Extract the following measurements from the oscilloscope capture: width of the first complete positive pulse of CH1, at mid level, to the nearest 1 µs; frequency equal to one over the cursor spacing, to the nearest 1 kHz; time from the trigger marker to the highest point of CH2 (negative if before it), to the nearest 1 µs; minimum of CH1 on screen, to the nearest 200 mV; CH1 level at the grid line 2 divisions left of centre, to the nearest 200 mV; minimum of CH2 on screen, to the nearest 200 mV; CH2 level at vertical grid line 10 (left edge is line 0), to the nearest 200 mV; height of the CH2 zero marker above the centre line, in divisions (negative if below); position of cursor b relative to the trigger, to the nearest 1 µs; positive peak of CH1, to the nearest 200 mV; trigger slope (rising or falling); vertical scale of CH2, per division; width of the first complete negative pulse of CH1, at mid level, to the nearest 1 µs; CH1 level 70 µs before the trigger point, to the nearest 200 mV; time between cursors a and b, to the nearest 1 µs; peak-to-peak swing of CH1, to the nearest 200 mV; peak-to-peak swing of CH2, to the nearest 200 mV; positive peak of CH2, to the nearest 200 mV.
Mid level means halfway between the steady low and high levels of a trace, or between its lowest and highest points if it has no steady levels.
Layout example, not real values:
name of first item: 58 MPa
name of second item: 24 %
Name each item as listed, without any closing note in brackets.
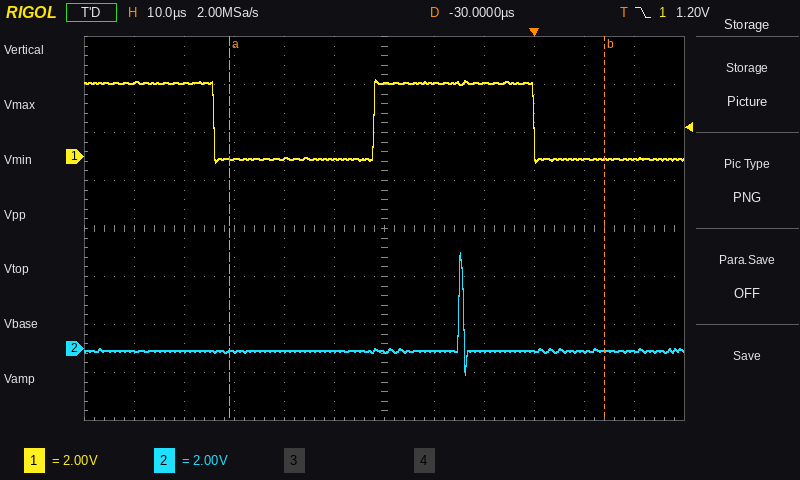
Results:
width of the first complete positive pulse of CH1, at mid level, to the nearest 1 µs: 32 µs
frequency equal to one over the cursor spacing, to the nearest 1 kHz: 13 kHz
time from the trigger marker to the highest point of CH2 (negative if before it), to the nearest 1 µs: -15 µs
minimum of CH1 on screen, to the nearest 200 mV: -200 mV
CH1 level at the grid line 2 divisions left of centre, to the nearest 200 mV: 0.0 V
minimum of CH2 on screen, to the nearest 200 mV: -1.0 V
CH2 level at vertical grid line 10 (left edge is line 0), to the nearest 200 mV: -200 mV
height of the CH2 zero marker above the centre line, in divisions: -2.5 div
position of cursor b relative to the trigger, to the nearest 1 µs: +14 µs
positive peak of CH1, to the nearest 200 mV: 3.2 V
trigger slope: falling
vertical scale of CH2, per division: 2 V
width of the first complete negative pulse of CH1, at mid level, to the nearest 1 µs: 32 µs
CH1 level 70 µs before the trigger point, to the nearest 200 mV: 3.0 V
time between cursors a and b, to the nearest 1 µs: 75 µs
peak-to-peak swing of CH1, to the nearest 200 mV: 3.4 V
peak-to-peak swing of CH2, to the nearest 200 mV: 5.0 V
positive peak of CH2, to the nearest 200 mV: 4.0 V
